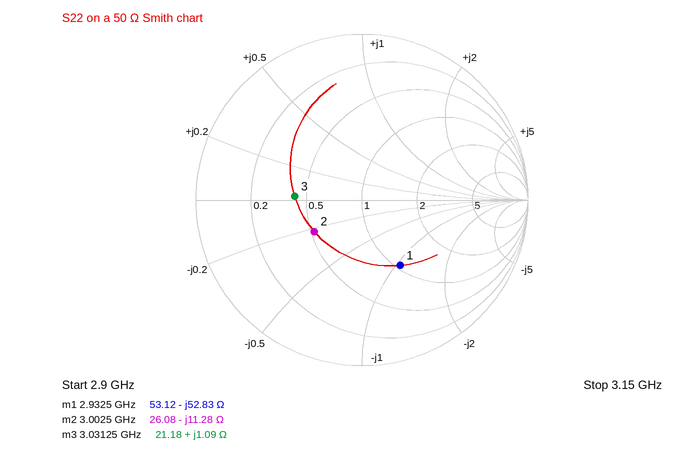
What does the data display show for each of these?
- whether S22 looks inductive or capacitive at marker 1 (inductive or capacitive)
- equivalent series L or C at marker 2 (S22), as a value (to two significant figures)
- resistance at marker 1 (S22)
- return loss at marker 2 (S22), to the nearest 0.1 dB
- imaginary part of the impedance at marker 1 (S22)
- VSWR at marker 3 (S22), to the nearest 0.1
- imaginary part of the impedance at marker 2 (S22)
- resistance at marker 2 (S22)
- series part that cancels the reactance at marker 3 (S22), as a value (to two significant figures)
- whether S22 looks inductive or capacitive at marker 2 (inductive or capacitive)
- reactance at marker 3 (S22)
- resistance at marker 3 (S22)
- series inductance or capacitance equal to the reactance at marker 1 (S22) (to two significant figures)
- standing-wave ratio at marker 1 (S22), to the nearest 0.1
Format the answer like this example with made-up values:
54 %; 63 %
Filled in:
capacitive; 4.7 pF; 53.12 Ω; 9.3 dB; -52.83 Ω; 2.4; -11.28 Ω; 26.08 Ω; 48 pF; capacitive; +1.09 Ω; 21.18 Ω; 1.0 pF; 2.7
